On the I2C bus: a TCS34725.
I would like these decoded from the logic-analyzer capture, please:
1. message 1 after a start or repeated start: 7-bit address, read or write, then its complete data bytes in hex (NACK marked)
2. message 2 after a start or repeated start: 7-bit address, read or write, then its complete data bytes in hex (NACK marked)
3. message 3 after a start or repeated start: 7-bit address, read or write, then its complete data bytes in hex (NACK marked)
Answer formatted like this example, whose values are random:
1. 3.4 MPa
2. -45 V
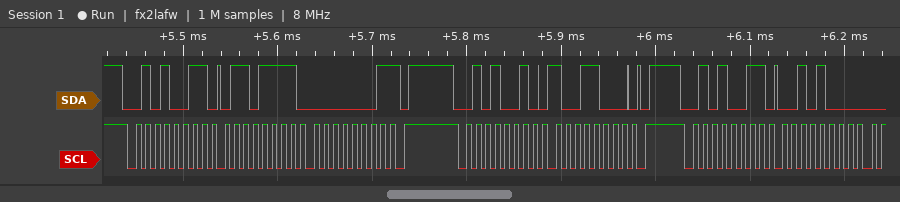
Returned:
1. 0x29 read: 6F 01 NACK
2. 0x29 write: 98
3. 0x29 read: 28
